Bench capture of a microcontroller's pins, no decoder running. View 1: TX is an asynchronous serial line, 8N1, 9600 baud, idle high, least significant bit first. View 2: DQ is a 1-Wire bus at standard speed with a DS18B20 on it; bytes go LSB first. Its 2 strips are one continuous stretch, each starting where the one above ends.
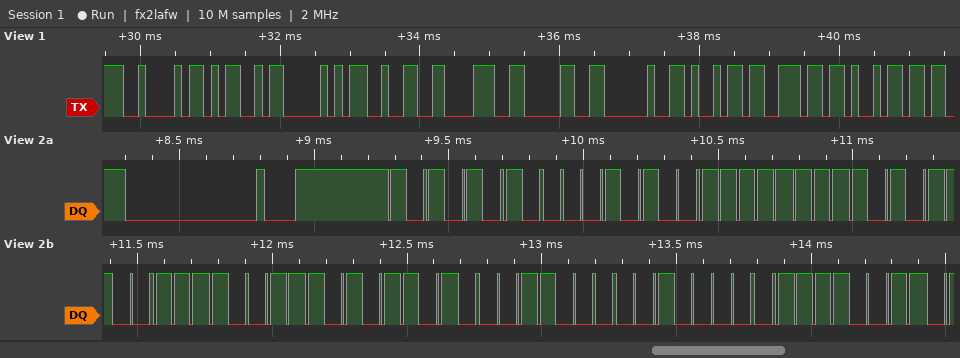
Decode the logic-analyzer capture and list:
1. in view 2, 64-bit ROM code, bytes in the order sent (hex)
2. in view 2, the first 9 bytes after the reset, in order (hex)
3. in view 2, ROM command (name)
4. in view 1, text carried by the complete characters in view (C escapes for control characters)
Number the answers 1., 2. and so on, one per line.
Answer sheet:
1. 28 FF 35 CF B5 18 04 CF
2. 55 28 FF 35 CF B5 18 04 CF
3. Match ROM
4. "BMP280 ini"
